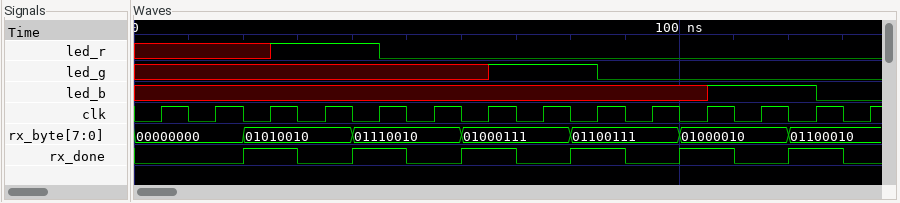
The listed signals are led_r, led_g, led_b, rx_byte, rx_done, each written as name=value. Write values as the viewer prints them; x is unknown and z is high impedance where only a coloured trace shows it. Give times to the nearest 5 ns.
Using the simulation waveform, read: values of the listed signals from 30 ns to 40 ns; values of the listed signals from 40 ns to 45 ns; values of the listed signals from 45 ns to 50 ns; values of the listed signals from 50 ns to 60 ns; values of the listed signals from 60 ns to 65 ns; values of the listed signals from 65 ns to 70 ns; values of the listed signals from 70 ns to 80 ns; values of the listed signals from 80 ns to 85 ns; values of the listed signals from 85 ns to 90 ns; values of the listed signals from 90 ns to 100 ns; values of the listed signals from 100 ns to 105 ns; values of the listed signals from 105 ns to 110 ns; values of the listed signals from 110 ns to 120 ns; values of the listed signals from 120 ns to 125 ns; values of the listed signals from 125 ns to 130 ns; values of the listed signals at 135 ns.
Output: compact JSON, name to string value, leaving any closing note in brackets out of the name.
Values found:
{"values of the listed signals from 30 ns to 40 ns": "led_r=1, led_g=x, led_b=x, rx_byte=01010010, rx_done=0", "values of the listed signals from 40 ns to 45 ns": "led_r=1, led_g=x, led_b=x, rx_byte=01110010, rx_done=1", "values of the listed signals from 45 ns to 50 ns": "led_r=0, led_g=x, led_b=x, rx_byte=01110010, rx_done=1", "values of the listed signals from 50 ns to 60 ns": "led_r=0, led_g=x, led_b=x, rx_byte=01110010, rx_done=0", "values of the listed signals from 60 ns to 65 ns": "led_r=0, led_g=x, led_b=x, rx_byte=01000111, rx_done=1", "values of the listed signals from 65 ns to 70 ns": "led_r=0, led_g=1, led_b=x, rx_byte=01000111, rx_done=1", "values of the listed signals from 70 ns to 80 ns": "led_r=0, led_g=1, led_b=x, rx_byte=01000111, rx_done=0", "values of the listed signals from 80 ns to 85 ns": "led_r=0, led_g=1, led_b=x, rx_byte=01100111, rx_done=1", "values of the listed signals from 85 ns to 90 ns": "led_r=0, led_g=0, led_b=x, rx_byte=01100111, rx_done=1", "values of the listed signals from 90 ns to 100 ns": "led_r=0, led_g=0, led_b=x, rx_byte=01100111, rx_done=0", "values of the listed signals from 100 ns to 105 ns": "led_r=0, led_g=0, led_b=x, rx_byte=01000010, rx_done=1", "values of the listed signals from 105 ns to 110 ns": "led_r=0, led_g=0, led_b=1, rx_byte=01000010, rx_done=1", "values of the listed signals from 110 ns to 120 ns": "led_r=0, led_g=0, led_b=1, rx_byte=01000010, rx_done=0", "values of the listed signals from 120 ns to 125 ns": "led_r=0, led_g=0, led_b=1, rx_byte=01100010, rx_done=1", "values of the listed signals from 125 ns to 130 ns": "led_r=0, led_g=0, led_b=0, rx_byte=01100010, rx_done=1", "values of the listed signals at 135 ns": "led_r=0, led_g=0, led_b=0, rx_byte=01100010, rx_done=0"}
